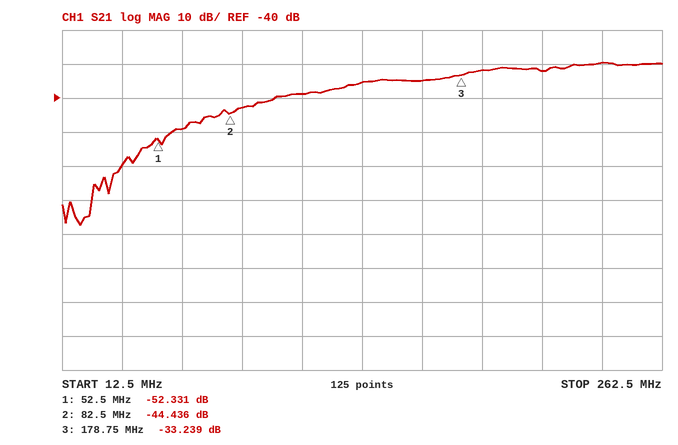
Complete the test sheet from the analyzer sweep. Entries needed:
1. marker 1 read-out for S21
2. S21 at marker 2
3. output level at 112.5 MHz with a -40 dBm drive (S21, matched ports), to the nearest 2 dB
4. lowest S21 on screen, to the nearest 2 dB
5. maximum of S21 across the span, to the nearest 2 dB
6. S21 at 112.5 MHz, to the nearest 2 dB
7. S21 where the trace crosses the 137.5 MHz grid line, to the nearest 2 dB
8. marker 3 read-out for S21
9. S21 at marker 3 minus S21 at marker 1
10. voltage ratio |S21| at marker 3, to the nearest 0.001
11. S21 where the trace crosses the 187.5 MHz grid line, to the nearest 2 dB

-52.331 dB
-44.436 dB
-78 dBm
-78 dB
-30 dB
-38 dB
-36 dB
-33.239 dB
19.092 dB
0.022
-32 dB
